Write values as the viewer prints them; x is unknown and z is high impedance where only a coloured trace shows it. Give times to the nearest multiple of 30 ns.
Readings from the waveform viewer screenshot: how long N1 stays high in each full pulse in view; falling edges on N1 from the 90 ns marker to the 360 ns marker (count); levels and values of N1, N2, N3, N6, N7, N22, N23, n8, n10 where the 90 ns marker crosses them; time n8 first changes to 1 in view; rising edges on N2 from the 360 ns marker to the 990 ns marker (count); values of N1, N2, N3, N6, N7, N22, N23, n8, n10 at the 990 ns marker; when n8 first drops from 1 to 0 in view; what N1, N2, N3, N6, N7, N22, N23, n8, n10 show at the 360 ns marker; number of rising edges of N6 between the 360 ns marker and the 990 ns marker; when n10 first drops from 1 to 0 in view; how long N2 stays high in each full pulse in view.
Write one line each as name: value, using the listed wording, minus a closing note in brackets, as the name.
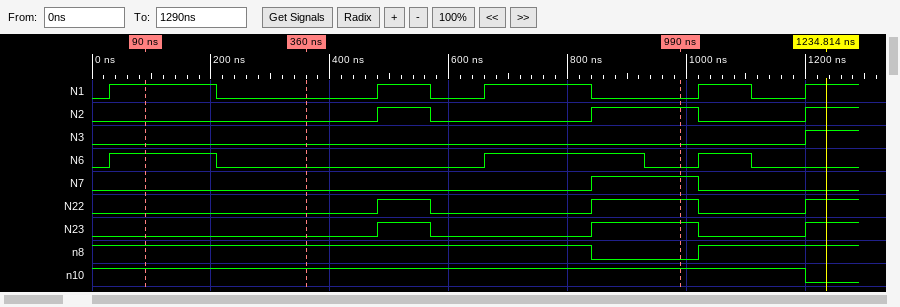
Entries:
how long N1 stays high in each full pulse in view: 180 ns, 90 ns, 180 ns, 90 ns
falling edges on N1 from the 90 ns marker to the 360 ns marker: 1
levels and values of N1, N2, N3, N6, N7, N22, N23, n8, n10 where the 90 ns marker crosses them: N1=1, N2=0, N3=0, N6=1, N7=0, N22=0, N23=0, n8=1, n10=1
time n8 first changes to 1 in view: 1020 ns
rising edges on N2 from the 360 ns marker to the 990 ns marker: 2
values of N1, N2, N3, N6, N7, N22, N23, n8, n10 at the 990 ns marker: N1=0, N2=1, N3=0, N6=0, N7=1, N22=1, N23=1, n8=0, n10=1
when n8 first drops from 1 to 0 in view: 840 ns
what N1, N2, N3, N6, N7, N22, N23, n8, n10 show at the 360 ns marker: N1=0, N2=0, N3=0, N6=0, N7=0, N22=0, N23=0, n8=1, n10=1
number of rising edges of N6 between the 360 ns marker and the 990 ns marker: 1
when n10 first drops from 1 to 0 in view: 1200 ns
how long N2 stays high in each full pulse in view: 90 ns, 180 ns
